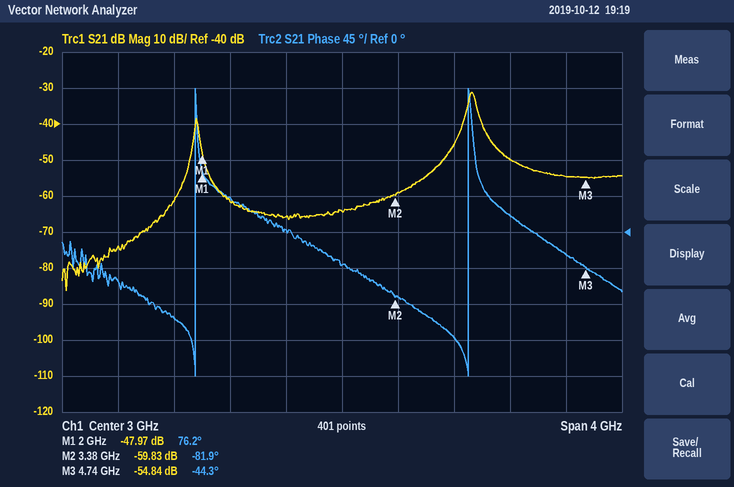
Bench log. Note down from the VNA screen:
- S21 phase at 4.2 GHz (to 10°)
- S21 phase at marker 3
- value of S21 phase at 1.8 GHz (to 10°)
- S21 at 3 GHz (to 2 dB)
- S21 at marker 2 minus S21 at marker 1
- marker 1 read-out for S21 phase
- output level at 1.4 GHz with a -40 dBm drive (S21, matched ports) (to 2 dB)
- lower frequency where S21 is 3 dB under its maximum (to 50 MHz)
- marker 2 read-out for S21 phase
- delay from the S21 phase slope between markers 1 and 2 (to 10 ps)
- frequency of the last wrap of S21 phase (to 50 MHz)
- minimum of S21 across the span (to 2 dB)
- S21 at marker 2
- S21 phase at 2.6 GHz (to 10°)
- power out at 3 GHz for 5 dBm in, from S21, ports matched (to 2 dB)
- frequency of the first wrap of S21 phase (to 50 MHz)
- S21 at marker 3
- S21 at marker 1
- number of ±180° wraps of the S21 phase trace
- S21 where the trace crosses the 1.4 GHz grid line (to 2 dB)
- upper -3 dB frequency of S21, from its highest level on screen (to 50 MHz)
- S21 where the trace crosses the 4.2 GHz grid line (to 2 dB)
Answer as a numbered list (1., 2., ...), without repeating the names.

1. 20°
2. -44.3°
3. -110°
4. -64 dB
5. -11.86 dB
6. 76.2°
7. -114 dBm
8. 3.90 GHz
9. -81.9°
10. 320 ps
11. 3.90 GHz
12. -86 dB
13. -59.83 dB
14. 0°
15. -60 dBm
16. 1.95 GHz
17. -54.84 dB
18. -47.97 dB
19. 2
20. -74 dB
21. 3.95 GHz
22. -50 dB
